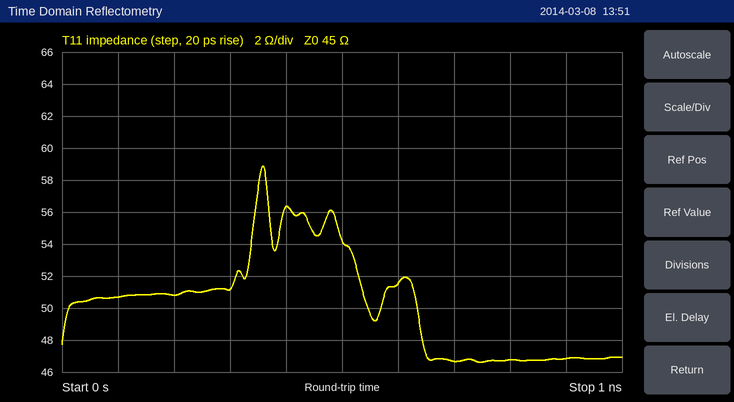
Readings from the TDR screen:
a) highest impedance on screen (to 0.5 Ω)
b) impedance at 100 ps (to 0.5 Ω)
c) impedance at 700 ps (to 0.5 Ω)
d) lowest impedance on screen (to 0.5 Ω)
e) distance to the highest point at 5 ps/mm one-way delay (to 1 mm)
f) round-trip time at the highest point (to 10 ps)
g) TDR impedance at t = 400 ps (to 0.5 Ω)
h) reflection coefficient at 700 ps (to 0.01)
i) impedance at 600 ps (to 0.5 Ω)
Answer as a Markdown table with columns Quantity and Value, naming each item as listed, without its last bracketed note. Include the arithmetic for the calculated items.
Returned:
| Quantity | Value |
|---|---|
| highest impedance on screen | 59.0 Ω |
| impedance at 100 ps | 50.5 Ω |
| impedance at 700 ps | 46.5 Ω |
| lowest impedance on screen | 46.5 Ω |
| distance to the highest point at 5 ps/mm one-way delay | 360 ps / 2 / 5 ps/mm ≈ 36 mm |
| round-trip time at the highest point | 360 ps |
| TDR impedance at t = 400 ps | 56.5 Ω |
| reflection coefficient at 700 ps | (46.5 − 45)/(46.5 + 45) ≈ +0.02 |
| impedance at 600 ps | 51.5 Ω |
